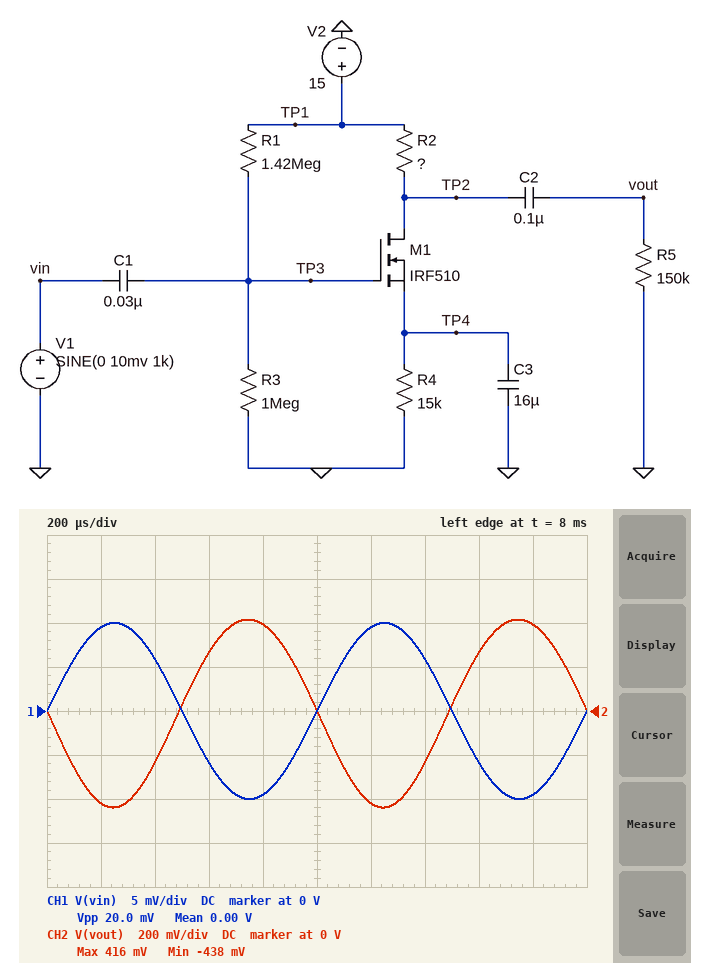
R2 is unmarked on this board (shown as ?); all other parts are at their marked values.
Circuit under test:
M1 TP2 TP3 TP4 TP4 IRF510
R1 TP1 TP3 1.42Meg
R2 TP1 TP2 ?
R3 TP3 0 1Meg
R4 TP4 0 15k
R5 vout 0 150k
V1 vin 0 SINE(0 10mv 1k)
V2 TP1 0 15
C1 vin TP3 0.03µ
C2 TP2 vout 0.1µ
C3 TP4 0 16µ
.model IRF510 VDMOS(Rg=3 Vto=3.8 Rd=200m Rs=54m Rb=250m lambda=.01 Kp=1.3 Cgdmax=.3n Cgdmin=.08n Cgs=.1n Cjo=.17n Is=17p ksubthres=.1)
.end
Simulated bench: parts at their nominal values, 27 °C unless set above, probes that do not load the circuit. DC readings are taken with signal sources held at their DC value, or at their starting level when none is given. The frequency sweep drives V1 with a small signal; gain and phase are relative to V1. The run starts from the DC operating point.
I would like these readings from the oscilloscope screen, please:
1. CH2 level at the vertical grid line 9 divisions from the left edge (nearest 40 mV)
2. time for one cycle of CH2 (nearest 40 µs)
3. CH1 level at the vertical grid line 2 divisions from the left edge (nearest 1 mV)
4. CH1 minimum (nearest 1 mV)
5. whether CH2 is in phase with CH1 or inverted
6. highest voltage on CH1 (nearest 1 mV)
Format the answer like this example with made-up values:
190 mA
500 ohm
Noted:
400 mV
1.00 ms
6 mV
-10 mV
inverted
10 mV
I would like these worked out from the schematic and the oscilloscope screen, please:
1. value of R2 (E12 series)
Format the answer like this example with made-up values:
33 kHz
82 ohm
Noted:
18 kΩ
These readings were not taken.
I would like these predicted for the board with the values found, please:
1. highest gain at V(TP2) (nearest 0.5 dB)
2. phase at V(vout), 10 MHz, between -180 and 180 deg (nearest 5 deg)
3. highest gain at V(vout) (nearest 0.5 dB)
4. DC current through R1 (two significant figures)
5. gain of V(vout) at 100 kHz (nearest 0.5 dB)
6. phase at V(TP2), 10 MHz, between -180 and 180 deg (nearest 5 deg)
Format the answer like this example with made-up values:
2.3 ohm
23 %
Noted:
32.5 dB
25 deg
32.5 dB
6.2 µA
28.5 dB
25 deg
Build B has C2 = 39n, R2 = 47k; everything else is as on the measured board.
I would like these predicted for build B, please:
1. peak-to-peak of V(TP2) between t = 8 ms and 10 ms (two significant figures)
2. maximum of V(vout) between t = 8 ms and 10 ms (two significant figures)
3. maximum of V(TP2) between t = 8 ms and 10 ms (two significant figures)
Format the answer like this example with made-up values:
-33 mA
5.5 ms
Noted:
1.3 V
680 mV
7.6 V
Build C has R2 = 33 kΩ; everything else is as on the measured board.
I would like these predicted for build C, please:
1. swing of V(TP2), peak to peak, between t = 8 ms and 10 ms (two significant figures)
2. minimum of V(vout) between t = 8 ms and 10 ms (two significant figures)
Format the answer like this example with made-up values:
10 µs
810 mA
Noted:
1.3 V
-640 mV
